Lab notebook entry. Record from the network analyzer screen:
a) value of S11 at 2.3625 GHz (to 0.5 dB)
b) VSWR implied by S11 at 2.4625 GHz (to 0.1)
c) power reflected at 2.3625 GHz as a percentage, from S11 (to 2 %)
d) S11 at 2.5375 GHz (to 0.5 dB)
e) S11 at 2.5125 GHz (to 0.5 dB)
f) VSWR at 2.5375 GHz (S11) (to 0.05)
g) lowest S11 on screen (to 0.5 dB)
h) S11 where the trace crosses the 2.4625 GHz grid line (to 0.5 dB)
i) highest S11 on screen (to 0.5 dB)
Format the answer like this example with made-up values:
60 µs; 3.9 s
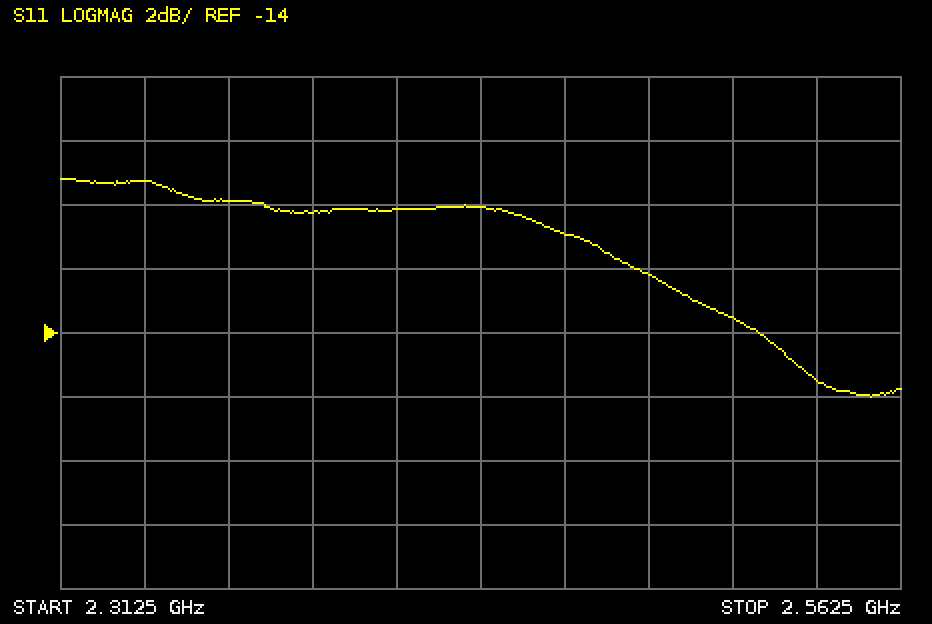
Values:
-10.0 dB; 1.8; 10 %; -15.5 dB; -13.5 dB; 1.40; -16.0 dB; -11.0 dB; -9.0 dB
